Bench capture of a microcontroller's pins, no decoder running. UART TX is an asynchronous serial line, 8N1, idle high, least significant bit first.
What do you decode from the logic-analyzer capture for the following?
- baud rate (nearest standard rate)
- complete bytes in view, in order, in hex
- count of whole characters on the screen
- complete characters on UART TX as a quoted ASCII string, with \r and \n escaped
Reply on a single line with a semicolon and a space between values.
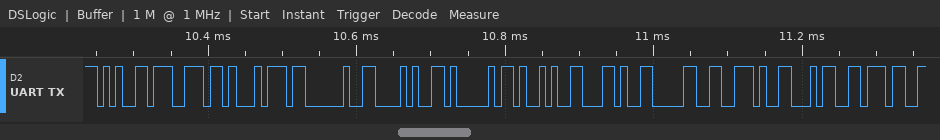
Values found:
115200 baud; 65 6E 74 20 28 41 29 2C 30 2E 34 37; 12; "ent (A),0.47"
